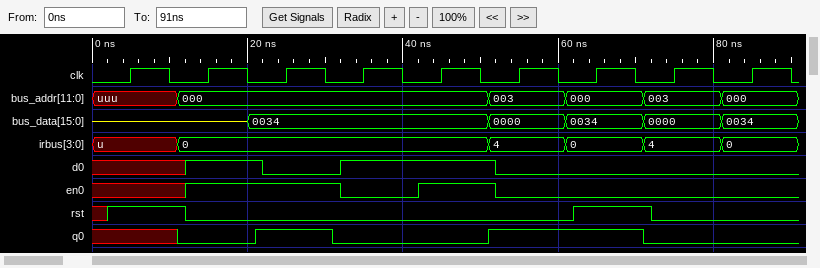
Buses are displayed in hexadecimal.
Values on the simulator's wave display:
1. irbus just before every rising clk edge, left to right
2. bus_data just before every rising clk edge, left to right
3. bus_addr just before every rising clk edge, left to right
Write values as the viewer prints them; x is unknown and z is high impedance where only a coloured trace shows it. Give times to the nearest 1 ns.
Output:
u, 0, 0, 0, 0, 4, 0, 4, 0
z, z, 0034, 0034, 0034, 0000, 0034, 0000, 0034
uuu, 000, 000, 000, 000, 003, 000, 003, 000
